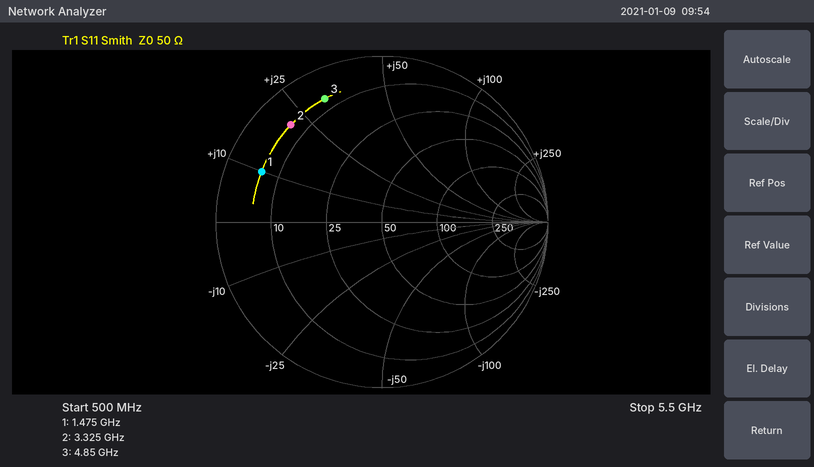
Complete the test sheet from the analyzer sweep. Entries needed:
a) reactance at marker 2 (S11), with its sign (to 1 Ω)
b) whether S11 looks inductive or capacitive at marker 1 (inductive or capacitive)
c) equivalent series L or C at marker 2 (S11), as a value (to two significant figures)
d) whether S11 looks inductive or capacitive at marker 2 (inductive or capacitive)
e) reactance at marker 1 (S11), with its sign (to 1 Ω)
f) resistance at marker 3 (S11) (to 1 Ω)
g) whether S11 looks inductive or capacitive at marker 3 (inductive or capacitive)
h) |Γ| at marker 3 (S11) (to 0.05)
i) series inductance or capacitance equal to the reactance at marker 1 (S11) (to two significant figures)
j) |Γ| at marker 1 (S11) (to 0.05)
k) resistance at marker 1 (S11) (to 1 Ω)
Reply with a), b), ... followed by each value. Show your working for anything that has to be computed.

a) +21 Ω
b) inductive
c) L = 21 Ω/(2π × 3.325 GHz) ≈ 1.0 nH
d) inductive
e) +10 Ω
f) 7 Ω
g) inductive
h) 0.80
i) L = 10 Ω/(2π × 1.475 GHz) ≈ 1.1 nH
j) 0.80
k) 6 Ω
